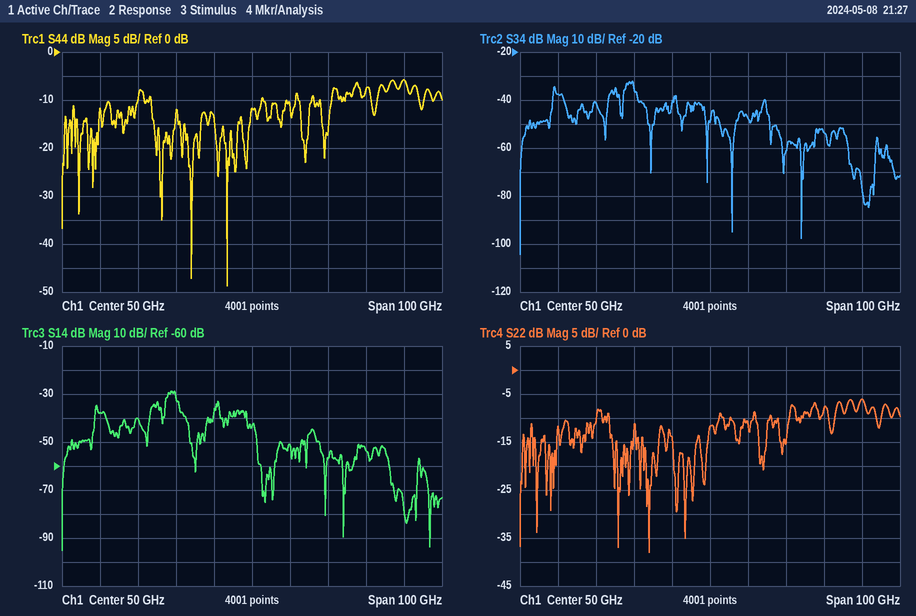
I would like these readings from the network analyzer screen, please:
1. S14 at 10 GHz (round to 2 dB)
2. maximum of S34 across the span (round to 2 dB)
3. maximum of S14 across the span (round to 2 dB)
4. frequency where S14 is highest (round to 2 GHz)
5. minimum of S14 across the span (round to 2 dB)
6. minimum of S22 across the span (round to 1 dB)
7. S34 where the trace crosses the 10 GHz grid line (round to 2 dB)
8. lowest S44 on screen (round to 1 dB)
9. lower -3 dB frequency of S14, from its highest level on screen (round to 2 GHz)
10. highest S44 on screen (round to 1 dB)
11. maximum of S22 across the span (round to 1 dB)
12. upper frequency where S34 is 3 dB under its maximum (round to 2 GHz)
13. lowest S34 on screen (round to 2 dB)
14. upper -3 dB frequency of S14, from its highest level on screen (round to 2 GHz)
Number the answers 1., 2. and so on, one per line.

1. -38 dB
2. -32 dB
3. -28 dB
4. 28 GHz
5. -96 dB
6. -38 dB
7. -38 dB
8. -49 dB
9. 28 GHz
10. -6 dB
11. -6 dB
12. 30 GHz
13. -104 dB
14. 30 GHz
